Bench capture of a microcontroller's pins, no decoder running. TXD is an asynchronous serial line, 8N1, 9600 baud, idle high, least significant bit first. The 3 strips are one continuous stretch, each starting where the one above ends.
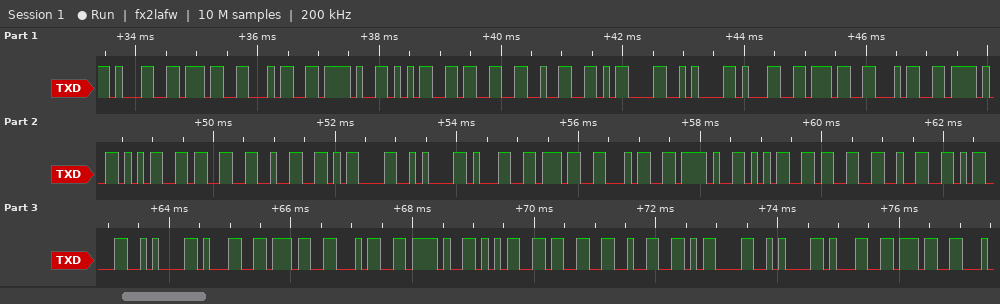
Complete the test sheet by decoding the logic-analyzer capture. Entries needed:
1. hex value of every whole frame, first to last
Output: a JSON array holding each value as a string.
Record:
["31 37 34 2F 35 33 32 0D 0A 31 37 34 2F 35 33 32 0D 0A 31 37 34 2F 35 33 32 0D 0A 31 37 34 2F 35 33 32 0D 0A 31 37"]
